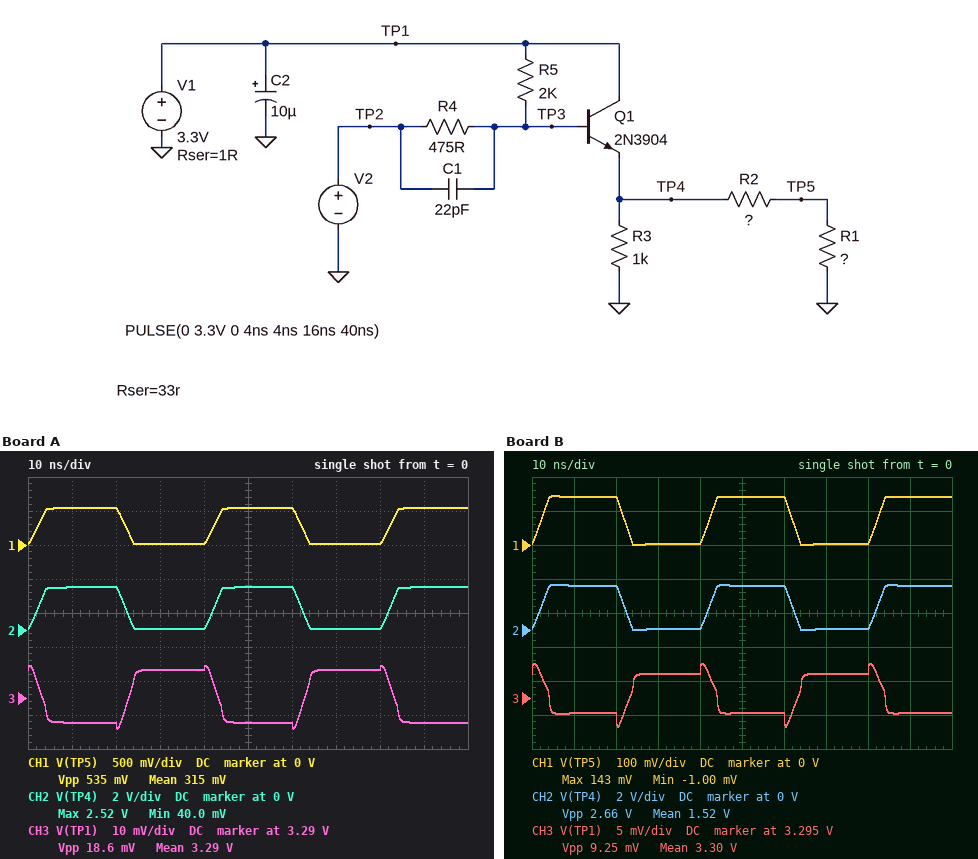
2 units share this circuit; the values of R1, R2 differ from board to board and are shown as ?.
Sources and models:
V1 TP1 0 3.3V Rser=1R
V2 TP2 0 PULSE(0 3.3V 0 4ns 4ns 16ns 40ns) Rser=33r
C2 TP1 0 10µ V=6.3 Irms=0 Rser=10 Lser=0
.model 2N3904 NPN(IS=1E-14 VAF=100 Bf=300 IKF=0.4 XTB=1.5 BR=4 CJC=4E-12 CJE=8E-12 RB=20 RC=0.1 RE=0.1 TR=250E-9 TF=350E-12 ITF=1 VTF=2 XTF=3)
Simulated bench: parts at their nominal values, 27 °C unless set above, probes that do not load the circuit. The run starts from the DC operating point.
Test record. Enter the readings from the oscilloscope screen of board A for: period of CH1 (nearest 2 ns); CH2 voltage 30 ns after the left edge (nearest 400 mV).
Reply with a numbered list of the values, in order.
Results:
1. 40 ns
2. 0 V
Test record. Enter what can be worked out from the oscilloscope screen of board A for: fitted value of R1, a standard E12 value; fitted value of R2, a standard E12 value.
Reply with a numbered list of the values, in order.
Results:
1. 33 Ω
2. 120 Ω
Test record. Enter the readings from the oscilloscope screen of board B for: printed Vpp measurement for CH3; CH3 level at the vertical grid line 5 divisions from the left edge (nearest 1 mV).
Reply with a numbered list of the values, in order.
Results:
1. 9.25 mV
2. 3.293 V
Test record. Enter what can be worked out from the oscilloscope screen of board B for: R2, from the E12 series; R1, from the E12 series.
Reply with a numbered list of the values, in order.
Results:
1. 470 Ω
2. 27 Ω
